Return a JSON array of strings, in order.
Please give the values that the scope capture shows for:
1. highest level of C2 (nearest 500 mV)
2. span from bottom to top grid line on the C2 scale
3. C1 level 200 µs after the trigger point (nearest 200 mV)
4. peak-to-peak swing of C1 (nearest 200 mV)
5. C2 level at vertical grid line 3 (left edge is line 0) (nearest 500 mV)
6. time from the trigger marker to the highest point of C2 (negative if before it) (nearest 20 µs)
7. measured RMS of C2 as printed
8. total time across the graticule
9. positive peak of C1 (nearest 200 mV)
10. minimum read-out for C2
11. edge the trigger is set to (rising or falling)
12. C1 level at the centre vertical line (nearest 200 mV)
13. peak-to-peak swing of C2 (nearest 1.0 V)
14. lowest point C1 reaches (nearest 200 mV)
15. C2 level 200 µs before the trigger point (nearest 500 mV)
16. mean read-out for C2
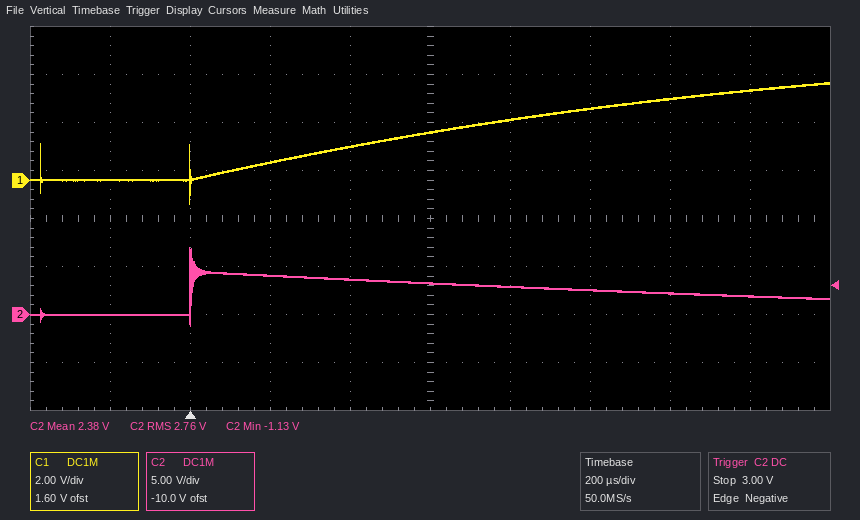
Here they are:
["7.0 V", "40 V", "800 mV", "5.0 V", "4.0 V", "0 µs", "2.76 V", "2 ms", "4.0 V", "-1.13 V", "falling", "2.0 V", "8.0 V", "-1.0 V", "0.0 V", "2.38 V"]
